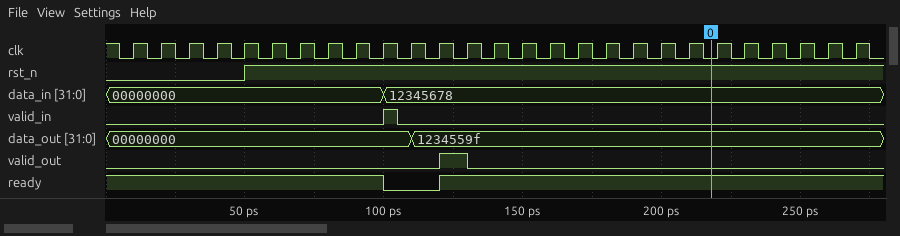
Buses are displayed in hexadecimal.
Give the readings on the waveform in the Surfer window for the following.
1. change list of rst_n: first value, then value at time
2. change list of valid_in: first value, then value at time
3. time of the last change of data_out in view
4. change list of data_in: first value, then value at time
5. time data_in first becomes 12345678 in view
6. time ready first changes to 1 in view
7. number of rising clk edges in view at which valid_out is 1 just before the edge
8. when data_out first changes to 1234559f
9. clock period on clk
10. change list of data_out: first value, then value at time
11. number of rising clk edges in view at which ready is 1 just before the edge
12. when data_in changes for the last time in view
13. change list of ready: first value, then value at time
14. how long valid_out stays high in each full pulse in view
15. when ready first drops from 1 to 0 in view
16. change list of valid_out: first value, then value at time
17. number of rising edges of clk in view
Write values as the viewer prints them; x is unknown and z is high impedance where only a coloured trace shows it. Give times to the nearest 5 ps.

0, 1 at 50 ps
0, 1 at 100 ps, 0 at 105 ps
110 ps
00000000, 12345678 at 100 ps
100 ps
120 ps
1
110 ps
10 ps
00000000, 1234559f at 110 ps
25
100 ps
1, 0 at 100 ps, 1 at 120 ps
10 ps
100 ps
0, 1 at 120 ps, 0 at 130 ps
27
